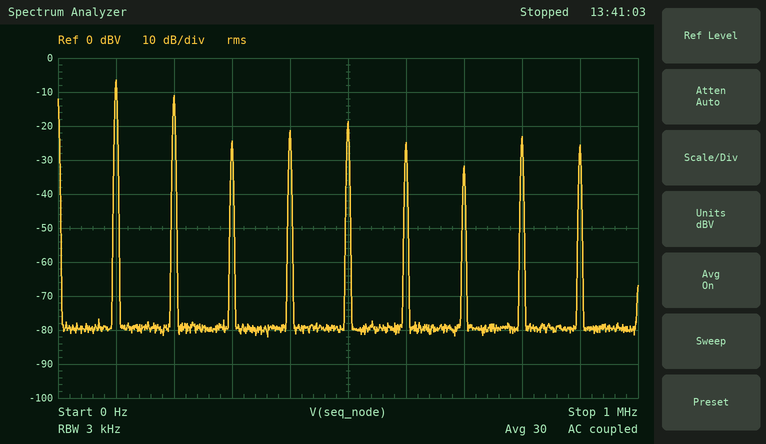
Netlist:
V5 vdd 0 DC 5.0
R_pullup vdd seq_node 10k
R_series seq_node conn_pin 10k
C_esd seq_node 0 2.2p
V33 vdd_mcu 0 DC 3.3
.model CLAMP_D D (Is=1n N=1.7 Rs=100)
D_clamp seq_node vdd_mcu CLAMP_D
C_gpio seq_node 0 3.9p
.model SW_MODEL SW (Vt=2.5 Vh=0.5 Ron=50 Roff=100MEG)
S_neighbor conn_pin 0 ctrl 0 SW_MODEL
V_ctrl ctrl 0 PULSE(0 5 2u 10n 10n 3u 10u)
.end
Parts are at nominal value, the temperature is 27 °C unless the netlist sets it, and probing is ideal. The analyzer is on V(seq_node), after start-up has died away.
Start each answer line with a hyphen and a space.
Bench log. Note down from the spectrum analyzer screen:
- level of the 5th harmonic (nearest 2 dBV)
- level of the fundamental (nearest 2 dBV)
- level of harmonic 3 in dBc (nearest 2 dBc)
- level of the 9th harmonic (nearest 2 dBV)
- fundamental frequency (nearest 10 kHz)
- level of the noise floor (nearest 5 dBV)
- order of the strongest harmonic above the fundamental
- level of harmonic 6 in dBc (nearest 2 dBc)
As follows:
- -18 dBV
- -6 dBV
- -18 dBc
- -26 dBV
- 100 kHz
- -80 dBV
- 2
- -18 dBc
